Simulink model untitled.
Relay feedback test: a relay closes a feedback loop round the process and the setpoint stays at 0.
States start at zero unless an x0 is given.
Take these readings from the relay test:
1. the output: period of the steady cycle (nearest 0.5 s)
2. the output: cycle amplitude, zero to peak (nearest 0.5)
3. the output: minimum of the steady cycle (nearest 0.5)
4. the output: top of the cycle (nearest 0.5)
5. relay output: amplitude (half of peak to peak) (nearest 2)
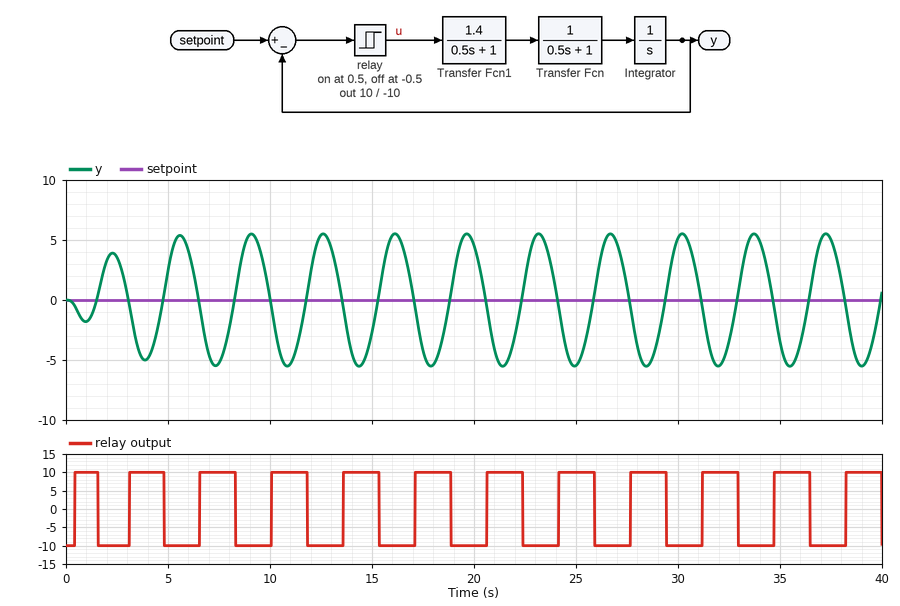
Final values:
3.5 s
5.5
-5.5
5.5
10
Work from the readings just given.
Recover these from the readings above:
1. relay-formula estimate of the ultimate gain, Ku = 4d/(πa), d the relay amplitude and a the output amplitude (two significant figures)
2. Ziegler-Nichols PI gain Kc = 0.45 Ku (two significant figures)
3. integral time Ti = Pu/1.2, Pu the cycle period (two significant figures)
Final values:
2.3
1.0
2.9 s
